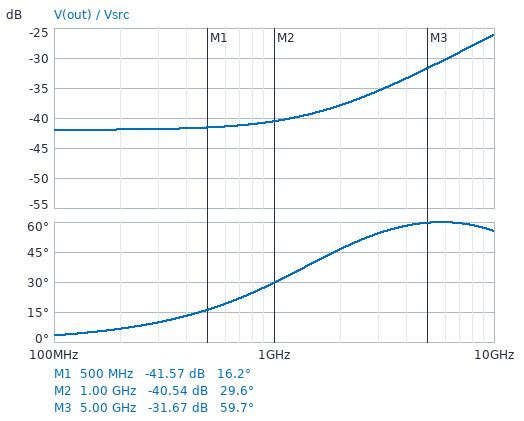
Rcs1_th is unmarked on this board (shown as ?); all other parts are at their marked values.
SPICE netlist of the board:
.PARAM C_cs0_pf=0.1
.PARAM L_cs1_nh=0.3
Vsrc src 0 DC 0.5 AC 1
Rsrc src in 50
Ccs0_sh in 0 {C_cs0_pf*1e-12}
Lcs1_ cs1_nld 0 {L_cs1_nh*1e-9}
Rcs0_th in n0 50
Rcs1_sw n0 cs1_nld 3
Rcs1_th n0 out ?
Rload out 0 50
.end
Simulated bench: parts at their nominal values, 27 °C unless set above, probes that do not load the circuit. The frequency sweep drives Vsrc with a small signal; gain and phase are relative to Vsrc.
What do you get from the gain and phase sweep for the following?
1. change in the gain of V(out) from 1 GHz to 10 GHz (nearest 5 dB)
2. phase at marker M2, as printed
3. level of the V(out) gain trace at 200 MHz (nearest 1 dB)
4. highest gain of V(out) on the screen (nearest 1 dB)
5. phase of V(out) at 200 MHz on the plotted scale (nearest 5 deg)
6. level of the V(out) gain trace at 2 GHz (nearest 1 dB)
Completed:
15 dB
29.6 deg
-42 dB
-26 dB
5 deg
-38 dB
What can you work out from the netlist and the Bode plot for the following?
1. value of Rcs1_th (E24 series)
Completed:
130 Ω
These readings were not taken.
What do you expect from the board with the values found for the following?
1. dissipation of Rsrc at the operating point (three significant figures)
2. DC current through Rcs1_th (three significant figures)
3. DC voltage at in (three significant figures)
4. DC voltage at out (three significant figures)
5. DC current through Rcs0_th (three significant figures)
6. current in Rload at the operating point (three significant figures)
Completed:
1.18 mW
79.6 µA
257 mV
3.98 mV
4.86 mA
79.6 µA
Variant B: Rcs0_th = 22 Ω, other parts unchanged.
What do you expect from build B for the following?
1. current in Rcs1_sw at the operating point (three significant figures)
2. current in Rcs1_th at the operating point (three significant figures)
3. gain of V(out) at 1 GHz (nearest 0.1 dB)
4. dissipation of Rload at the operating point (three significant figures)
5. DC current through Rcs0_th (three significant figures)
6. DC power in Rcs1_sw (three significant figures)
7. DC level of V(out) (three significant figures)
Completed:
6.56 mA
109 µA
-37.8 dB
598 nW
6.67 mA
129 µW
5.47 mV
